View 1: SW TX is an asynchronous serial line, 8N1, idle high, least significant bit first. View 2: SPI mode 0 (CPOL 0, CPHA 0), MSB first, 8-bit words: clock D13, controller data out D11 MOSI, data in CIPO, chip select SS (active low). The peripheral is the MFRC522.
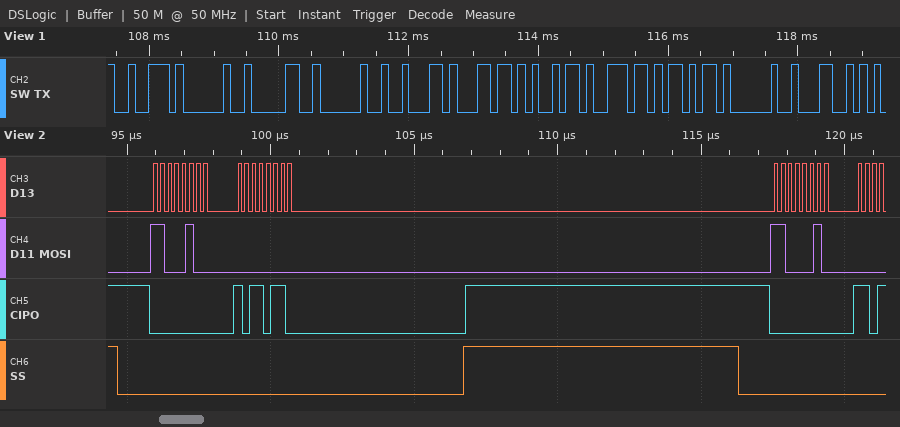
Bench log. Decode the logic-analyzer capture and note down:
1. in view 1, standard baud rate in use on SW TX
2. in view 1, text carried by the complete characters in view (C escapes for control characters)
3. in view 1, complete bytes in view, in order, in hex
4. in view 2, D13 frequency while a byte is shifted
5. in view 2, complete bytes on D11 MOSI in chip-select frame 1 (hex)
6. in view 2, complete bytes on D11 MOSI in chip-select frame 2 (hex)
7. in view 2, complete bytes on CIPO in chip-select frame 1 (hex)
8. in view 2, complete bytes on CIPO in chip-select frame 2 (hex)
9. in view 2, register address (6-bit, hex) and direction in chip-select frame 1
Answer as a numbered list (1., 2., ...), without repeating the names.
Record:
1. 9600 baud
2. "r 0 blink L"
3. 72 20 30 20 62 6C 69 6E 6B 20 4C
4. 4 MHz
5. 0xC4 0x00
6. 0xC2
7. 0x00 0xB6
8. 0x00
9. 0x22 read
